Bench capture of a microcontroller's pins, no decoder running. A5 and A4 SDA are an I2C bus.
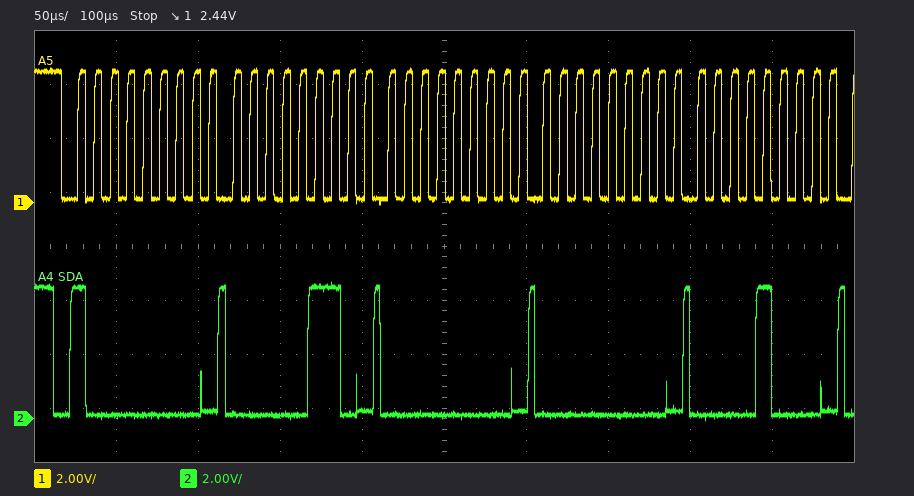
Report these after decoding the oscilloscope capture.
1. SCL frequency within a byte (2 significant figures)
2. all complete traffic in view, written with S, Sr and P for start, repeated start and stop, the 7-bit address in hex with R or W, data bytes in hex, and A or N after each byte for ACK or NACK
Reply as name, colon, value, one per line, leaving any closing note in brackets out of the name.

SCL frequency within a byte: 100 kHz
all complete traffic in view, written with S, Sr and P for start, repeated start and stop, the 7-bit address in hex with R or W, data bytes in hex, and A or N after each byte for ACK or NACK: S 40W A 06 A 00 A 00 A 08 A
